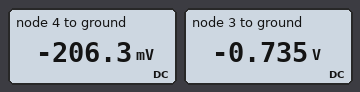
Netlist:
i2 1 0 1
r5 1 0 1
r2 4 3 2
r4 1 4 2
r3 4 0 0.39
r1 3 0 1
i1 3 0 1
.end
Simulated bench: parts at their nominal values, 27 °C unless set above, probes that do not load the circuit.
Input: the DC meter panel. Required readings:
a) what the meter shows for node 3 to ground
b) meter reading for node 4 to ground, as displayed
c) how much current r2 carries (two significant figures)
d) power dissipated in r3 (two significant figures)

-0.735 V
-206.3 mV
260 mA
110 mW
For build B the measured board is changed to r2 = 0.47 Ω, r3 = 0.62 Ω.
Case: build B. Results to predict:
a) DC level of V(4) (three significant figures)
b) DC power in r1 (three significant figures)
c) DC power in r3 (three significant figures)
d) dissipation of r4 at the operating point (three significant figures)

-386 mV
339 mW
240 mW
83.8 mW
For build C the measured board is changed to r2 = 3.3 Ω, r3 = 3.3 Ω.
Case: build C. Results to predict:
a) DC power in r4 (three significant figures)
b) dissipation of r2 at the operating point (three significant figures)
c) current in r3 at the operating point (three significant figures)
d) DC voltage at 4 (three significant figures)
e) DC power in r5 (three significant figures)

27.0 mW
21.7 mW
197 mA
-651 mV
781 mW
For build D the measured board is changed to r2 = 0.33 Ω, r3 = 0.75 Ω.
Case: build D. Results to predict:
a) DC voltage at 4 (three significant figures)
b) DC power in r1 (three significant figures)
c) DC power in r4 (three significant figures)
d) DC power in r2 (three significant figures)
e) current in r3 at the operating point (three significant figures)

-449 mV
343 mW
67.5 mW
56.7 mW
598 mA
